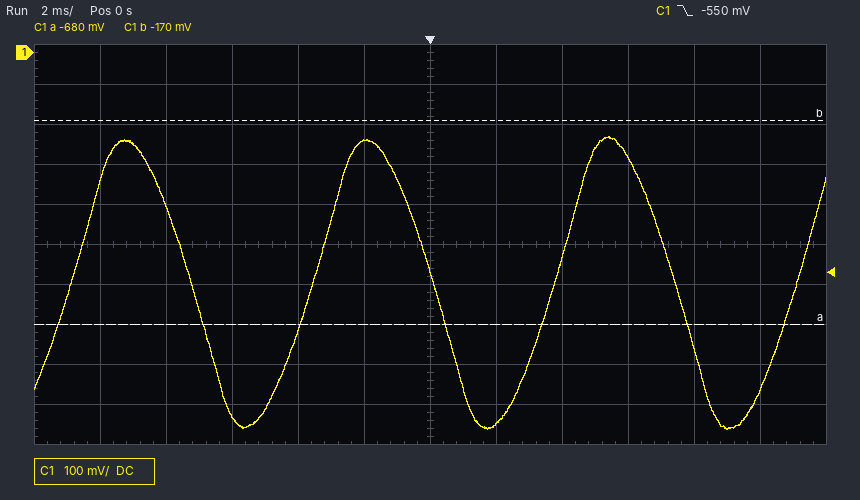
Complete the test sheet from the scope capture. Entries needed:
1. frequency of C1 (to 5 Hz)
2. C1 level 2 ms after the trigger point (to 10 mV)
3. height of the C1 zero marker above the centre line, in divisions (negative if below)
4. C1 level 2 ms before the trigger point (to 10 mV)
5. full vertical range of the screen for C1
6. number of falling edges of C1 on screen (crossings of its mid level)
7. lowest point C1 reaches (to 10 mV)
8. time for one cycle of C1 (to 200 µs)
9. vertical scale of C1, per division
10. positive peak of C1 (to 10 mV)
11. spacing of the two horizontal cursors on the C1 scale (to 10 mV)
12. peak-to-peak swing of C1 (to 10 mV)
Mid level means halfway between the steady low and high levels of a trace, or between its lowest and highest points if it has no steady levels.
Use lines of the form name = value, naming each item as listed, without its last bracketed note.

frequency of C1 = 135 Hz
C1 level 2 ms after the trigger point = -930 mV
height of the C1 zero marker above the centre line, in divisions = +4.8 div
C1 level 2 ms before the trigger point = -220 mV
full vertical range of the screen for C1 = 1 V
number of falling edges of C1 on screen = 3
lowest point C1 reaches = -940 mV
time for one cycle of C1 = 7.4 ms
vertical scale of C1, per division = 100 mV
positive peak of C1 = -210 mV
spacing of the two horizontal cursors on the C1 scale = 510 mV
peak-to-peak swing of C1 = 730 mV
